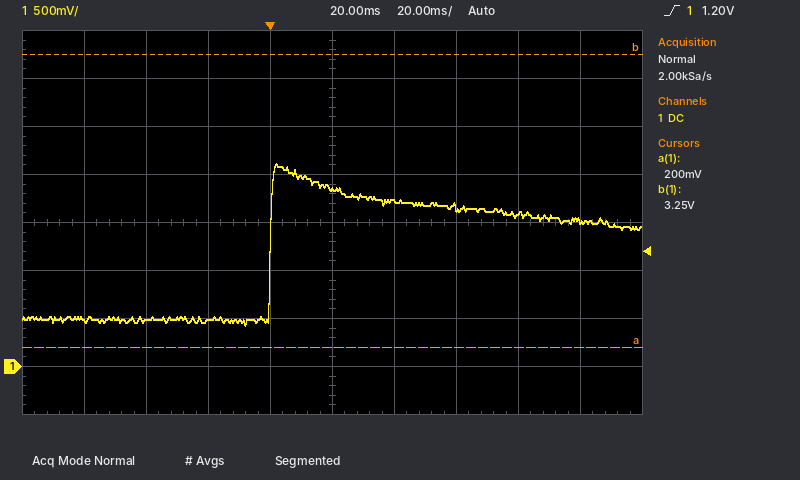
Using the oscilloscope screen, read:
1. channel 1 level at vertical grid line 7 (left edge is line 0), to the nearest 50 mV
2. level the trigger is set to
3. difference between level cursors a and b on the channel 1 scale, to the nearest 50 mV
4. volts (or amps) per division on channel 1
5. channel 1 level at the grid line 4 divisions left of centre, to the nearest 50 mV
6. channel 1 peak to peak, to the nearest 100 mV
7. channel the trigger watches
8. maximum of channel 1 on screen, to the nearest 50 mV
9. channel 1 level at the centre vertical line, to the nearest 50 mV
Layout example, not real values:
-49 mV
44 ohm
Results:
1.65 V
1.20 V
3.05 V
500 mV
500 mV
1.70 V
channel 1
2.10 V
1.85 V
